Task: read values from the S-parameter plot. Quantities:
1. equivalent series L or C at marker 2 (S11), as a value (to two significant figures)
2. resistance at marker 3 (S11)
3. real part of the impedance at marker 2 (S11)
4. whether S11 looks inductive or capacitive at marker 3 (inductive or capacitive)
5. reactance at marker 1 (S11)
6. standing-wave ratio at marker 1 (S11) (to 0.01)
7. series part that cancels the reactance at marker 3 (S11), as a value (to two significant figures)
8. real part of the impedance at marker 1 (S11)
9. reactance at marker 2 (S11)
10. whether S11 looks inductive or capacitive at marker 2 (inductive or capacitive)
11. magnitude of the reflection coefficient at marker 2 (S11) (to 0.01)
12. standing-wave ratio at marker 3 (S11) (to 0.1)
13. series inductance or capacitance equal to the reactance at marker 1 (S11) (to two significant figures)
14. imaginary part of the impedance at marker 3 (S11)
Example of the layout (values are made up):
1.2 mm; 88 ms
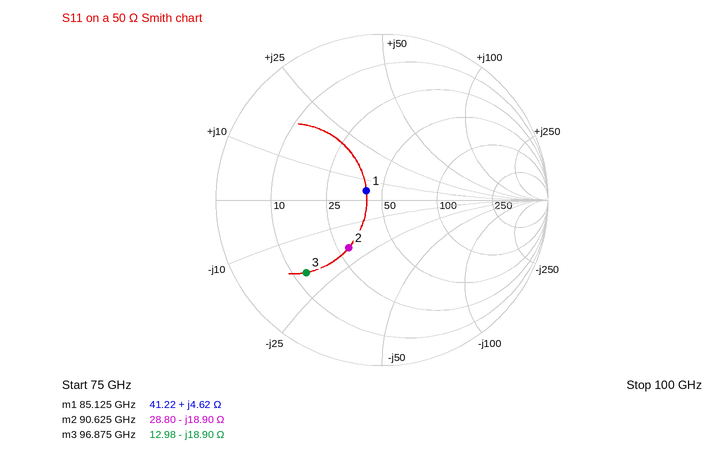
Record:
93 fF; 12.98 Ω; 28.80 Ω; capacitive; +4.62 Ω; 1.24; 31 pH; 41.22 Ω; -18.90 Ω; capacitive; 0.35; 4.4; 8.6 pH; -18.90 Ω
